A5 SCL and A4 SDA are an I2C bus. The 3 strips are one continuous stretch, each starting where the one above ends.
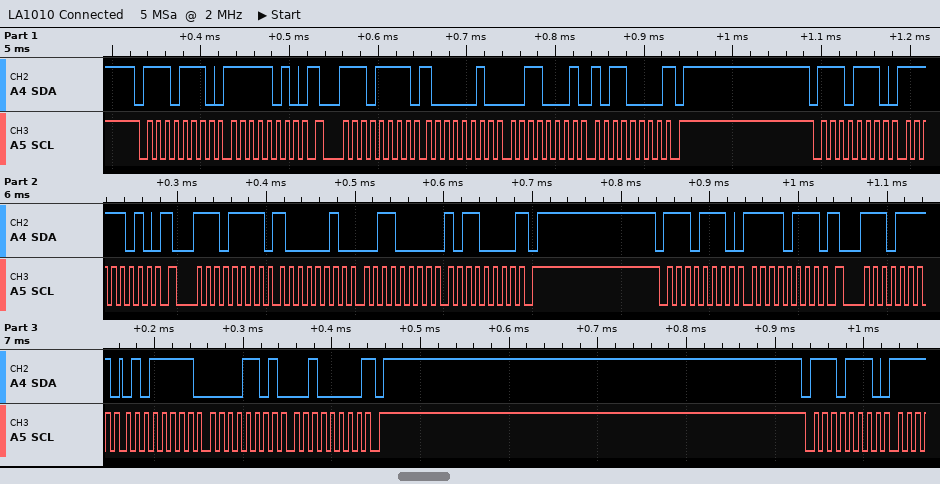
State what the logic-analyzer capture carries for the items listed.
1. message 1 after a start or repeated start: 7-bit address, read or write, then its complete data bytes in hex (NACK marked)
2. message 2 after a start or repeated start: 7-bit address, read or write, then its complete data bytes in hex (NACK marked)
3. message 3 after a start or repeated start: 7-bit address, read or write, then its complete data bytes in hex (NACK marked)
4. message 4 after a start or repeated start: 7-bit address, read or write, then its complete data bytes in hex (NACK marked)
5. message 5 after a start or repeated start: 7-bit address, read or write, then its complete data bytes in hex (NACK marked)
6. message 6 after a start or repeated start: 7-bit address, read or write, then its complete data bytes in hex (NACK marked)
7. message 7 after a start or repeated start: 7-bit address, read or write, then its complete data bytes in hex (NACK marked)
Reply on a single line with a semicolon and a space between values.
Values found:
0x77 write: FA; 0x77 read: 82 31 B0 NACK; 0x77 write: FA; 0x77 read: 82 30 B0 NACK; 0x77 write: F7; 0x77 read: 5F 0D 20 NACK; 0x77 write
